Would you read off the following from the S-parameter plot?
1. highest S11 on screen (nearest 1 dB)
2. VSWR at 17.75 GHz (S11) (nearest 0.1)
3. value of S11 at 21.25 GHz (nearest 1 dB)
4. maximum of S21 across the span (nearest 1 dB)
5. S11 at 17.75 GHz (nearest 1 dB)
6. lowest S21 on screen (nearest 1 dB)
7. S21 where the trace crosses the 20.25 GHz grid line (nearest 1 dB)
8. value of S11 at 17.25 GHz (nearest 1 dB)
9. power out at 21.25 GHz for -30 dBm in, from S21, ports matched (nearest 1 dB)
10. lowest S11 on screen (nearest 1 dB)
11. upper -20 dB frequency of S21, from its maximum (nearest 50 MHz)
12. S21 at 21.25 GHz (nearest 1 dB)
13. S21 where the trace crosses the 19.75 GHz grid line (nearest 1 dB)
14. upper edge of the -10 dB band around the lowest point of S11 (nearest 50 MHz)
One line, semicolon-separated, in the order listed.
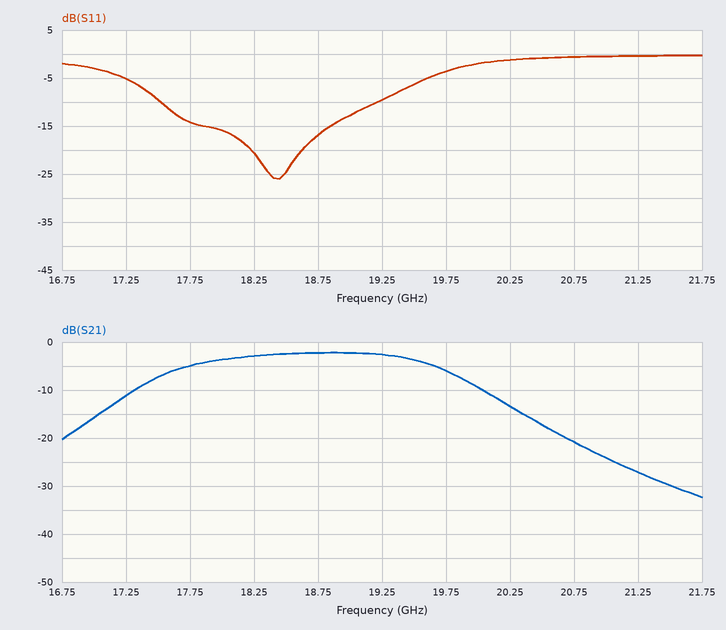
0 dB; 1.5; 0 dB; -2 dB; -14 dB; -32 dB; -13 dB; -5 dB; -57 dBm; -26 dB; 20.85 GHz; -27 dB; -6 dB; 19.20 GHz
